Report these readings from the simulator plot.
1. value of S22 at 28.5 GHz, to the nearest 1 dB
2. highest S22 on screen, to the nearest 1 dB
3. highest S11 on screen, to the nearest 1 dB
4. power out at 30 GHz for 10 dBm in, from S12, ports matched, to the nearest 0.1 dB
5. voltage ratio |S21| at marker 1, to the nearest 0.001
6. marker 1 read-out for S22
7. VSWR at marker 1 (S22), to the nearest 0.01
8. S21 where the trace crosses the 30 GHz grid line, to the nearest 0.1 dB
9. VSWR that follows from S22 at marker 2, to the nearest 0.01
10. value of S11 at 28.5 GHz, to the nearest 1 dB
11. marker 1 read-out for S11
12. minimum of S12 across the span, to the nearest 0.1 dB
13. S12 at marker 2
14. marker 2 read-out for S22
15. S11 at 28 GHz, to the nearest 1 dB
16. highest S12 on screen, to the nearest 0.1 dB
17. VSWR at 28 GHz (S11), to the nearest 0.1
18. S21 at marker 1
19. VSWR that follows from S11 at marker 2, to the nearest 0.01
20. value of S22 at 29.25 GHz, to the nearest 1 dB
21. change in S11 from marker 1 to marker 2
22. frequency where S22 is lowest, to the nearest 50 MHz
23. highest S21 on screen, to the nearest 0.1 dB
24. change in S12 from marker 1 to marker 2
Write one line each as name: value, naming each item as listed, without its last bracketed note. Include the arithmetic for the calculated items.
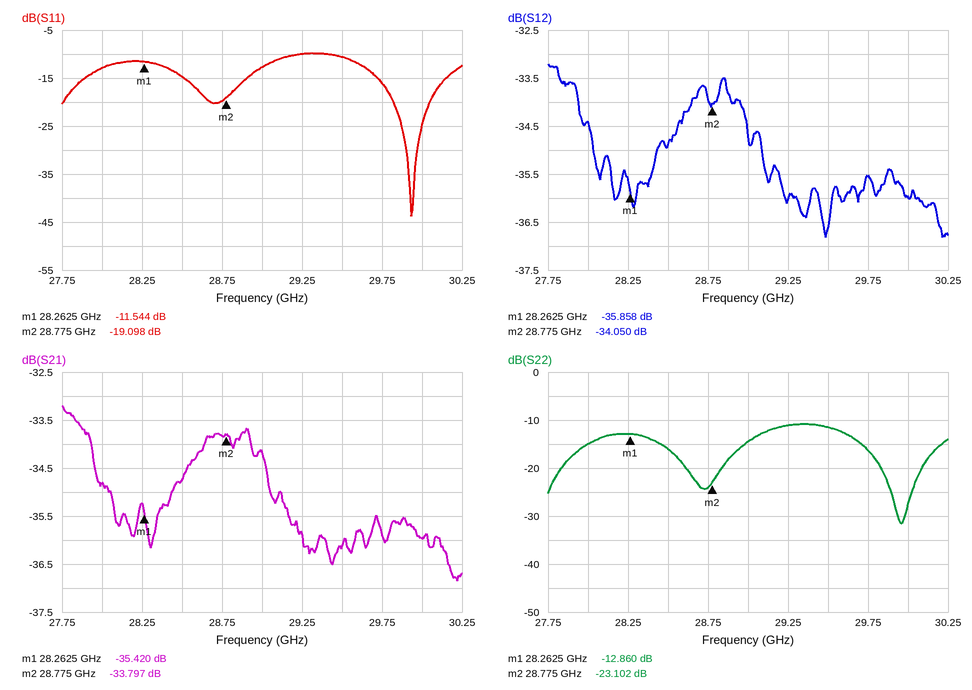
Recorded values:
value of S22 at 28.5 GHz, to the nearest 1 dB: -16 dB
highest S22 on screen, to the nearest 1 dB: -11 dB
highest S11 on screen, to the nearest 1 dB: -10 dB
power out at 30 GHz for 10 dBm in, from S12, ports matched, to the nearest 0.1 dB: 10 dBm + (-36.0 dB) = -26.0 dBm
voltage ratio |S21| at marker 1, to the nearest 0.001: 10^(-35.42/20) ≈ 0.017
marker 1 read-out for S22: -12.860 dB
VSWR at marker 1 (S22), to the nearest 0.01: (1 + 0.2275)/(1 − 0.2275) ≈ 1.59
S21 where the trace crosses the 30 GHz grid line, to the nearest 0.1 dB: -36.0 dB
VSWR that follows from S22 at marker 2, to the nearest 0.01: (1 + 0.0700)/(1 − 0.0700) ≈ 1.15
value of S11 at 28.5 GHz, to the nearest 1 dB: -15 dB
marker 1 read-out for S11: -11.544 dB
minimum of S12 across the span, to the nearest 0.1 dB: -36.8 dB
S12 at marker 2: -34.050 dB
marker 2 read-out for S22: -23.102 dB
S11 at 28 GHz, to the nearest 1 dB: -13 dB
highest S12 on screen, to the nearest 0.1 dB: -33.2 dB
VSWR at 28 GHz (S11), to the nearest 0.1: |Γ| = 10^(-13/20) = 0.2239; VSWR = (1 + 0.2239)/(1 − 0.2239) ≈ 1.6
S21 at marker 1: -35.420 dB
VSWR that follows from S11 at marker 2, to the nearest 0.01: (1 + 0.1109)/(1 − 0.1109) ≈ 1.25
value of S22 at 29.25 GHz, to the nearest 1 dB: -11 dB
change in S11 from marker 1 to marker 2: -19.098 − (-11.544) = -7.554 dB
frequency where S22 is lowest, to the nearest 50 MHz: 29.95 GHz
highest S21 on screen, to the nearest 0.1 dB: -33.2 dB
change in S12 from marker 1 to marker 2: -34.05 − (-35.858) = 1.808 dB
